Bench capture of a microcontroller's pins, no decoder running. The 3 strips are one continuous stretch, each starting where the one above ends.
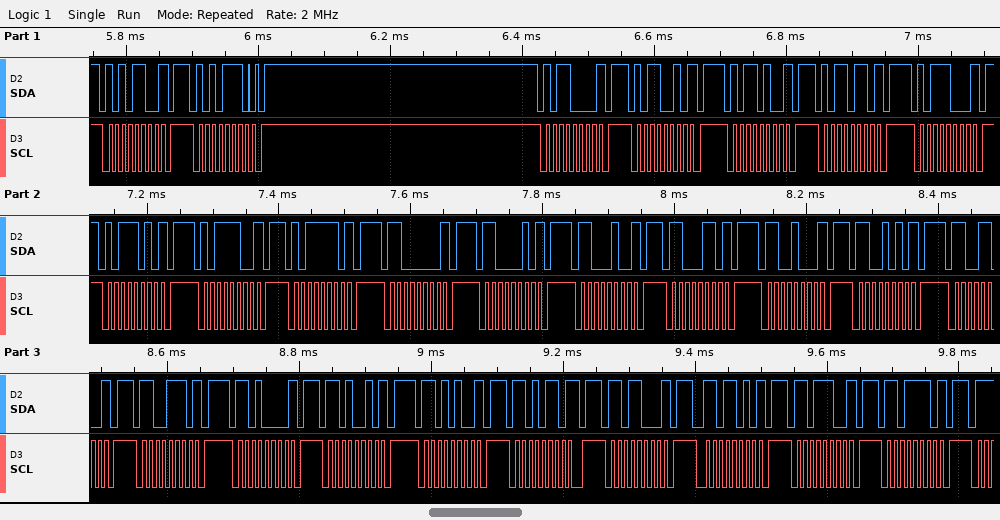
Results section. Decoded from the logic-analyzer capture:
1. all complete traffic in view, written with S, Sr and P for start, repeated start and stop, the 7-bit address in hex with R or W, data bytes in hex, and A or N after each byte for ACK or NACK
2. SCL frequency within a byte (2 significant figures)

S 56W N P S 57W A P S 58W N P S 59W N P S 5AW N P S 5BW N P S 5CW N P S 5DW N P S 5EW N P S 5FW N P S 60W N P S 61W N P S 62W N P S 63W N P S 64W N P S 65W N P S 66W N P S 67W N P S 68W N P S 69W N P S 6AW N P S 6BW N P S 6CW N P S 6DW N P S 6EW N P S 6FW N P
100 kHz
